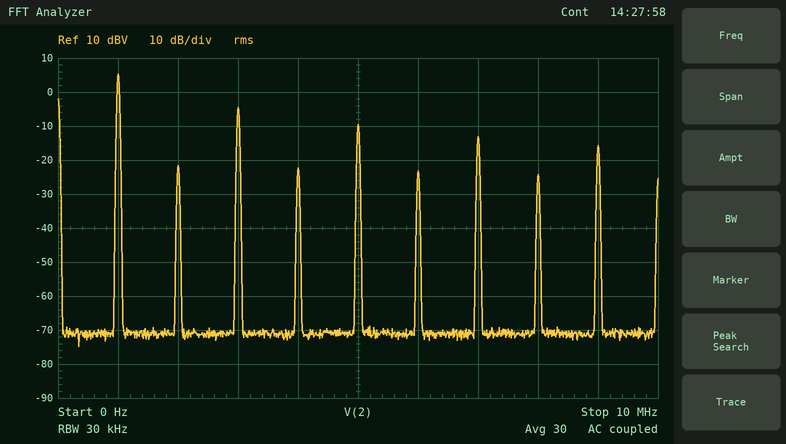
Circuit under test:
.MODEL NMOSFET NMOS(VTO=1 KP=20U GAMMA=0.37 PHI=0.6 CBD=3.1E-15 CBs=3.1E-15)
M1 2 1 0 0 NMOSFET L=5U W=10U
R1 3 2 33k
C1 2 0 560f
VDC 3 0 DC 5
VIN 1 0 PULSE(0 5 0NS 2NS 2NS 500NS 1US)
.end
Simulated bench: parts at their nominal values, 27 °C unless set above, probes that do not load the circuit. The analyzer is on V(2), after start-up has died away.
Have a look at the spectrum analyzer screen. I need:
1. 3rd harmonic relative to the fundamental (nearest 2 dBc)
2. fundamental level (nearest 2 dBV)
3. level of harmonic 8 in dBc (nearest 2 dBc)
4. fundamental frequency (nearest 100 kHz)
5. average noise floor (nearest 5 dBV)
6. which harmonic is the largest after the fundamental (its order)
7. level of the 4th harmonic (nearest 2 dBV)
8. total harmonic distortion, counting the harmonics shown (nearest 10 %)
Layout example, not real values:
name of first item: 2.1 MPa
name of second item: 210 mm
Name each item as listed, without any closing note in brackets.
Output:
3rd harmonic relative to the fundamental: -10 dBc
fundamental level: 6 dBV
level of harmonic 8 in dBc: -30 dBc
fundamental frequency: 1.0 MHz
average noise floor: -70 dBV
which harmonic is the largest after the fundamental: 3
level of the 4th harmonic: -22 dBV
total harmonic distortion, counting the harmonics shown: 40 %
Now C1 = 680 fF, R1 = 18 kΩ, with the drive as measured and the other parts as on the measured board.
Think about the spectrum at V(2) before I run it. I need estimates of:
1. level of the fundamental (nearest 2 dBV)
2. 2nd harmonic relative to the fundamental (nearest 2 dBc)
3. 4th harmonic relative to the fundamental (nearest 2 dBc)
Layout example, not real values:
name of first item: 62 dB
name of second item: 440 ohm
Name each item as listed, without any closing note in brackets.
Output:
level of the fundamental: 4 dBV
2nd harmonic relative to the fundamental: -32 dBc
4th harmonic relative to the fundamental: -32 dBc
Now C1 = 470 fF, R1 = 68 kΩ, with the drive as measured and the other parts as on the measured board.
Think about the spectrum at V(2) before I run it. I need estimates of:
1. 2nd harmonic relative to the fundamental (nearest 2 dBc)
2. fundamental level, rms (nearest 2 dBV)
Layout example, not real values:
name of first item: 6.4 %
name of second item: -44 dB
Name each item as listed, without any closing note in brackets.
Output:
2nd harmonic relative to the fundamental: -22 dBc
fundamental level, rms: 6 dBV
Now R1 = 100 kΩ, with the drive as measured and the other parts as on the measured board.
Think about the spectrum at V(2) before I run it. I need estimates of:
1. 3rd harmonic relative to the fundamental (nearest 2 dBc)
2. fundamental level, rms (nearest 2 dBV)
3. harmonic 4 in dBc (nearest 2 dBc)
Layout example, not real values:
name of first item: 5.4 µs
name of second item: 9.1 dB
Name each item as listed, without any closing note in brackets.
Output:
3rd harmonic relative to the fundamental: -12 dBc
fundamental level, rms: 6 dBV
harmonic 4 in dBc: -20 dBc
